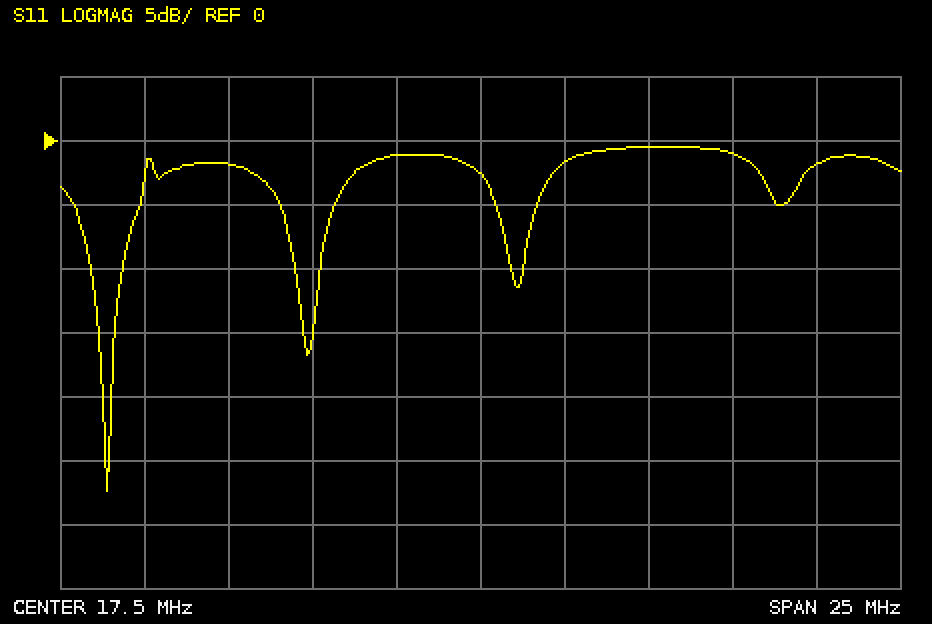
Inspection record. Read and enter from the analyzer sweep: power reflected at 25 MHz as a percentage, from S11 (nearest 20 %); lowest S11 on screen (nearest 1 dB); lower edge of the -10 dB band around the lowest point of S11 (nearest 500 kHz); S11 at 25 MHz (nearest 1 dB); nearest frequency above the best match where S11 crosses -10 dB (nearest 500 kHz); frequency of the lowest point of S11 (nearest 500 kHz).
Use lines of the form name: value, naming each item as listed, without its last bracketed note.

power reflected at 25 MHz as a percentage, from S11: 80 %
lowest S11 on screen: -27 dB
lower edge of the -10 dB band around the lowest point of S11: 6.0 MHz
S11 at 25 MHz: -1 dB
nearest frequency above the best match where S11 crosses -10 dB: 7.0 MHz
frequency of the lowest point of S11: 6.5 MHz
